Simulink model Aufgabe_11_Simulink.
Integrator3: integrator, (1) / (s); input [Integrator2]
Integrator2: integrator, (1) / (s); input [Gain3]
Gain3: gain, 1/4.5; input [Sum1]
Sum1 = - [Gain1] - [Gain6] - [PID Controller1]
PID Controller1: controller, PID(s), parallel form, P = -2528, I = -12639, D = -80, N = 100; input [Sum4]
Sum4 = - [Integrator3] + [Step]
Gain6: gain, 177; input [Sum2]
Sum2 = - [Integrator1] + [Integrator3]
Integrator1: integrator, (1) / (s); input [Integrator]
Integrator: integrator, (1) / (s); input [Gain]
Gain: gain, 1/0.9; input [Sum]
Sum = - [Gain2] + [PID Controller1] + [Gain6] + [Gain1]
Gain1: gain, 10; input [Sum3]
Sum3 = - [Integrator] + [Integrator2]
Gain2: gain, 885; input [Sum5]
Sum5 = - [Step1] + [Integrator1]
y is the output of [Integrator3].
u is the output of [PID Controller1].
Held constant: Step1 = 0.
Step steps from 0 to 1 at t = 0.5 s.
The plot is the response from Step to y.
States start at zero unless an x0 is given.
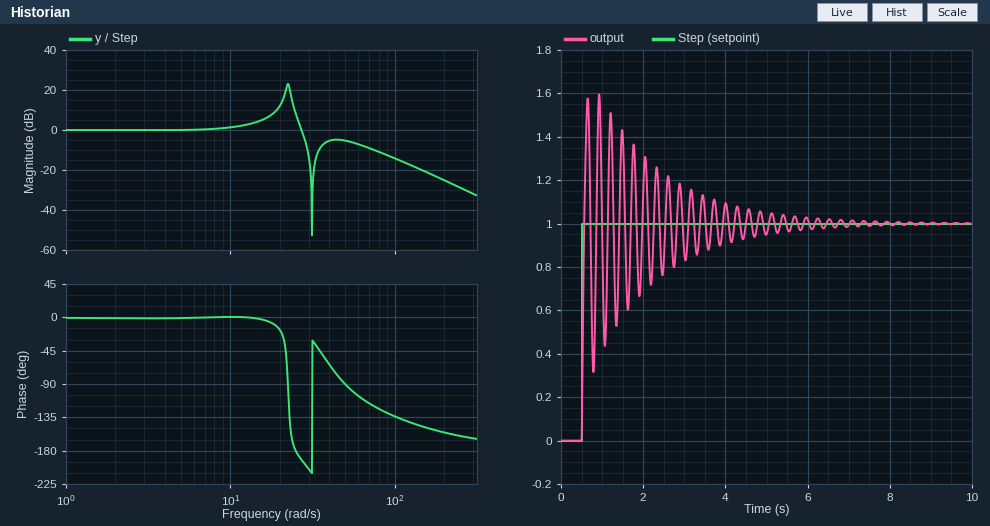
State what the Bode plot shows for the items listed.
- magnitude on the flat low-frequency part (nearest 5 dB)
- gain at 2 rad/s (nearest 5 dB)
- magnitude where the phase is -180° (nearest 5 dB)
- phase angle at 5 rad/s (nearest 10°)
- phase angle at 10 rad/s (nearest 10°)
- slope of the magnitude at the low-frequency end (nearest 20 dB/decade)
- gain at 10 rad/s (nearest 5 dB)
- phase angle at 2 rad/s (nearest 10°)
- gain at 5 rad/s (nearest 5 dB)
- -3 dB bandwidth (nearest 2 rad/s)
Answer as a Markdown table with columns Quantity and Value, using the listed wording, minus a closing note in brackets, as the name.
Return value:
| Quantity | Value |
|---|---|
| magnitude on the flat low-frequency part | 0 dB |
| gain at 2 rad/s | 0 dB |
| magnitude where the phase is -180° | 10 dB |
| phase angle at 5 rad/s | 0° |
| phase angle at 10 rad/s | 0° |
| slope of the magnitude at the low-frequency end | 0 dB/decade |
| gain at 10 rad/s | 0 dB |
| phase angle at 2 rad/s | 0° |
| gain at 5 rad/s | 0 dB |
| -3 dB bandwidth | 28 rad/s |
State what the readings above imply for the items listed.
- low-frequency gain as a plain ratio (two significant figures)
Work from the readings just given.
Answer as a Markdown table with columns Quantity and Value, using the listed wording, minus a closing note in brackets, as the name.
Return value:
| Quantity | Value |
|---|---|
| low-frequency gain as a plain ratio | 1.0 |
